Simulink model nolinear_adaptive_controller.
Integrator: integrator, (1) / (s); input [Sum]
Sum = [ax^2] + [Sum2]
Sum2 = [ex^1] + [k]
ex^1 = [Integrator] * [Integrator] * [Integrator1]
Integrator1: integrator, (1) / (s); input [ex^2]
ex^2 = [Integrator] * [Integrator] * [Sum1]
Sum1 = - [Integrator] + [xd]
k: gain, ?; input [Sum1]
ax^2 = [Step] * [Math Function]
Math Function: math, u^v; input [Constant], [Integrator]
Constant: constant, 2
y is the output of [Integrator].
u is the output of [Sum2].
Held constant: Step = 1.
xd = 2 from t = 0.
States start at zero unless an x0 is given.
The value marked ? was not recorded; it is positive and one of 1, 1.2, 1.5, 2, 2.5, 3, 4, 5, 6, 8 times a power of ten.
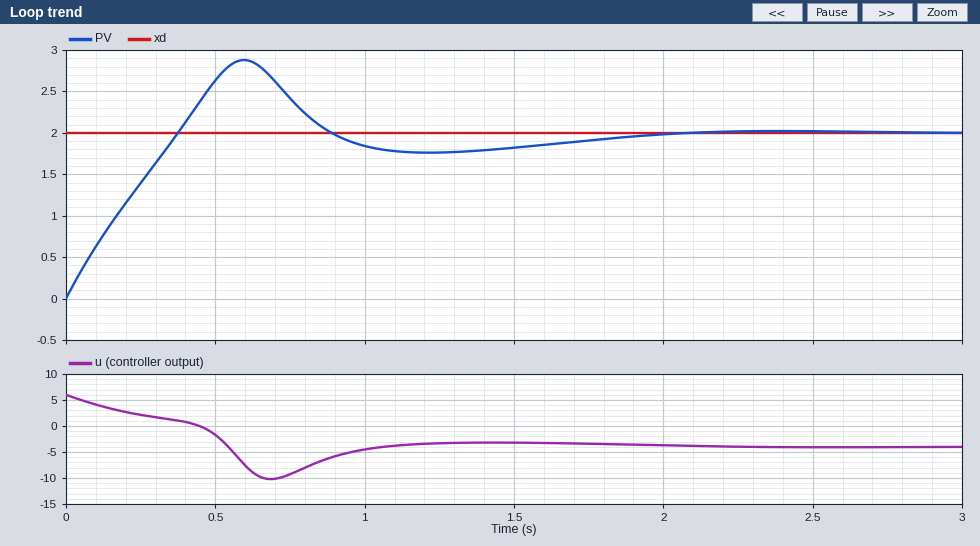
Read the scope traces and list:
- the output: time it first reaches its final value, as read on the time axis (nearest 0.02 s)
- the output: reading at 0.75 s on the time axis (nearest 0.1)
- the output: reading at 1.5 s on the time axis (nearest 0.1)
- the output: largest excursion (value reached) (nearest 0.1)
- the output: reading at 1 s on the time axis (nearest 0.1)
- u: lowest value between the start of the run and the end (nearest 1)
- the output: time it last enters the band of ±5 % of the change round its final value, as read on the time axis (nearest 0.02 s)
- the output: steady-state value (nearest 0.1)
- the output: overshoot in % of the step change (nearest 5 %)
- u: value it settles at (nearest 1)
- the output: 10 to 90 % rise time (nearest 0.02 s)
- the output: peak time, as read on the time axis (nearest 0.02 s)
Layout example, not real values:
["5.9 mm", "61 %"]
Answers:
["0.38 s", "2.4", "1.8", "2.9", "1.8", "-10", "1.72 s", "2.0", "45 %", "-4", "0.30 s", "0.60 s"]
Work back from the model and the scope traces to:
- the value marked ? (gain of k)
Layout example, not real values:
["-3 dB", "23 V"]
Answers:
["3"]
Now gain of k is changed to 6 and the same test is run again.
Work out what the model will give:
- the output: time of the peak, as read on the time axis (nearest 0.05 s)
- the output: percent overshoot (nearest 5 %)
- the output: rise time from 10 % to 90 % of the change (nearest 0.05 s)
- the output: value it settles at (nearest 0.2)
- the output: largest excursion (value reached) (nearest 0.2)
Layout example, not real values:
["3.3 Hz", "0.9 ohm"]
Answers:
["0.50 s", "30 %", "0.20 s", "2.0", "2.6"]
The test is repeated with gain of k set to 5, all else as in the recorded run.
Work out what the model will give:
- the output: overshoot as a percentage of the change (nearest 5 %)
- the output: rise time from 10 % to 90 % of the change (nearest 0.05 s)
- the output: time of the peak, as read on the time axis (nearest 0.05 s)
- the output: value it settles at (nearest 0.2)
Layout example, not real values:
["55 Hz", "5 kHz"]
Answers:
["35 %", "0.25 s", "0.50 s", "2.0"]
